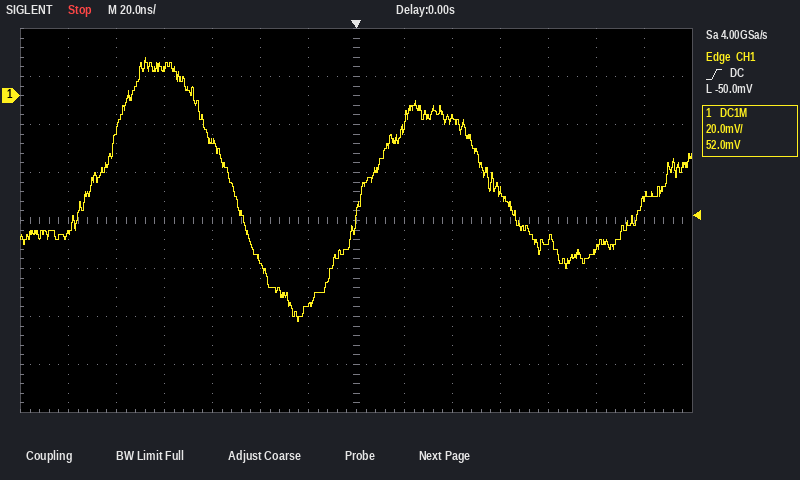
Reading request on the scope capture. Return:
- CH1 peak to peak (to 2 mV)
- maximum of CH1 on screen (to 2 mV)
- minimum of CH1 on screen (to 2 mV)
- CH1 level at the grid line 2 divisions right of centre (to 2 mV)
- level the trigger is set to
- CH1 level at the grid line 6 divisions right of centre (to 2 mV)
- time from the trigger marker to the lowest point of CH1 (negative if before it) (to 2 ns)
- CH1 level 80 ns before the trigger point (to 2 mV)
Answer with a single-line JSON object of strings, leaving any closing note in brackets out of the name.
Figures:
{"CH1 peak to peak": "110 mV", "maximum of CH1 on screen": "16 mV", "minimum of CH1 on screen": "-94 mV", "CH1 level at the grid line 2 divisions right of centre": "-10 mV", "level the trigger is set to": "-50.0 mV", "CH1 level at the grid line 6 divisions right of centre": "-42 mV", "time from the trigger marker to the lowest point of CH1 (negative if before it)": "-24 ns", "CH1 level 80 ns before the trigger point": "12 mV"}
